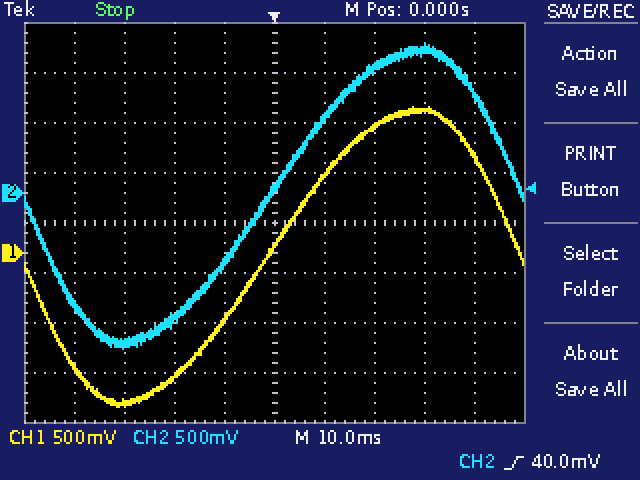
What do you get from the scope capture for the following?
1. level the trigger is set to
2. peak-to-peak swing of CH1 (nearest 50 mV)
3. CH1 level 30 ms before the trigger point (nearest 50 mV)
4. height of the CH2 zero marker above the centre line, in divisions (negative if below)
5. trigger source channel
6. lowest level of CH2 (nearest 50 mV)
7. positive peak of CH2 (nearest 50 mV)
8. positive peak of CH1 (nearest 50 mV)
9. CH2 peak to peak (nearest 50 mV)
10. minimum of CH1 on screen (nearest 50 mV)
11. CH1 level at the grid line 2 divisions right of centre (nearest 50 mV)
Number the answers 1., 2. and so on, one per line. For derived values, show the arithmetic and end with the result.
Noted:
1. 40.0 mV
2. 1.45 V − (-1.55 V) = 3.00 V
3. -1.50 V
4. +0.6 div
5. CH2
6. -1.55 V
7. 1.50 V
8. 1.45 V
9. 1.50 V − (-1.55 V) = 3.05 V
10. -1.55 V
11. 1.25 V
